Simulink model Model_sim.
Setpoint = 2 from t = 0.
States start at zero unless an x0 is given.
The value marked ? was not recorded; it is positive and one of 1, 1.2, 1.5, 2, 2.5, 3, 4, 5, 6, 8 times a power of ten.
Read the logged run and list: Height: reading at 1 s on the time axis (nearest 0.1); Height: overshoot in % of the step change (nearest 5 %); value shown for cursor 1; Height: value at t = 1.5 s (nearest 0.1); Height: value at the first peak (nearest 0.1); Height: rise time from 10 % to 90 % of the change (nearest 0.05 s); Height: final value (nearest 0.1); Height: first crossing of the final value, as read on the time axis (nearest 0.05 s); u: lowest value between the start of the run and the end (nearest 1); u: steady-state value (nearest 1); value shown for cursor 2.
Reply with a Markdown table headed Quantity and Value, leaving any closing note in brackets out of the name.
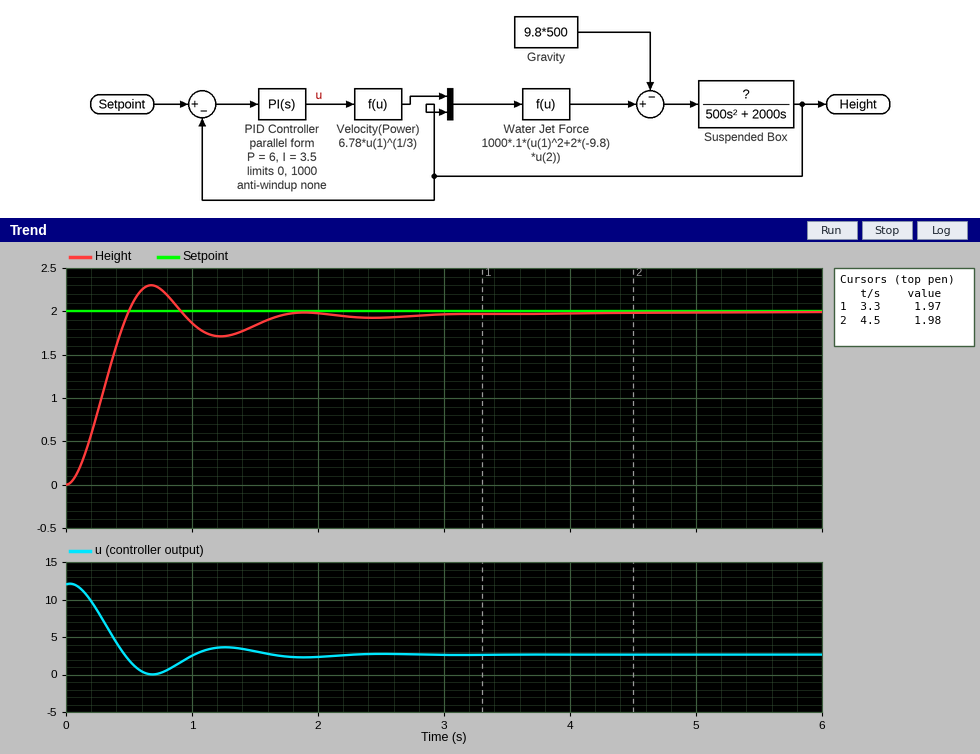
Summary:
| Quantity | Value |
|---|---|
| Height: reading at 1 s on the time axis | 1.9 |
| Height: overshoot in % of the step change | 15 % |
| value shown for cursor 1 | 1.97 |
| Height: value at t = 1.5 s | 1.8 |
| Height: value at the first peak | 2.3 |
| Height: rise time from 10 % to 90 % of the change | 0.35 s |
| Height: final value | 2.0 |
| Height: first crossing of the final value, as read on the time axis | 0.50 s |
| u: lowest value between the start of the run and the end | 0 |
| u: steady-state value | 3 |
| value shown for cursor 2 | 1.98 |
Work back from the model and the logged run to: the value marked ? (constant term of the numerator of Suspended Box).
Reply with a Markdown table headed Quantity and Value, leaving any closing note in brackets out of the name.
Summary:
| Quantity | Value |
|---|---|
| the value marked ? | 1 |
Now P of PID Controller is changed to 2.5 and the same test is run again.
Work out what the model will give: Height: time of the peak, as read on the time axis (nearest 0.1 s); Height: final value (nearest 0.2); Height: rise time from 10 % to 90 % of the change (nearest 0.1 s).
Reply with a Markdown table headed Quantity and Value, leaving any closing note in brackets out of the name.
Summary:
| Quantity | Value |
|---|---|
| Height: time of the peak, as read on the time axis | 1.1 s |
| Height: final value | 2.0 |
| Height: rise time from 10 % to 90 % of the change | 0.5 s |
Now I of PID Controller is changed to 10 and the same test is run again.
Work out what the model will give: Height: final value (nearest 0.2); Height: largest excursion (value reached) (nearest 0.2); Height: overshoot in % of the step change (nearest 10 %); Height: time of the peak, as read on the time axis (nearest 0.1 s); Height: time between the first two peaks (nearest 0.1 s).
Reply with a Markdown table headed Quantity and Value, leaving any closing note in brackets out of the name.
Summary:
| Quantity | Value |
|---|---|
| Height: final value | 2.0 |
| Height: largest excursion (value reached) | 2.8 |
| Height: overshoot in % of the step change | 40 % |
| Height: time of the peak, as read on the time axis | 0.7 s |
| Height: time between the first two peaks | 1.2 s |
